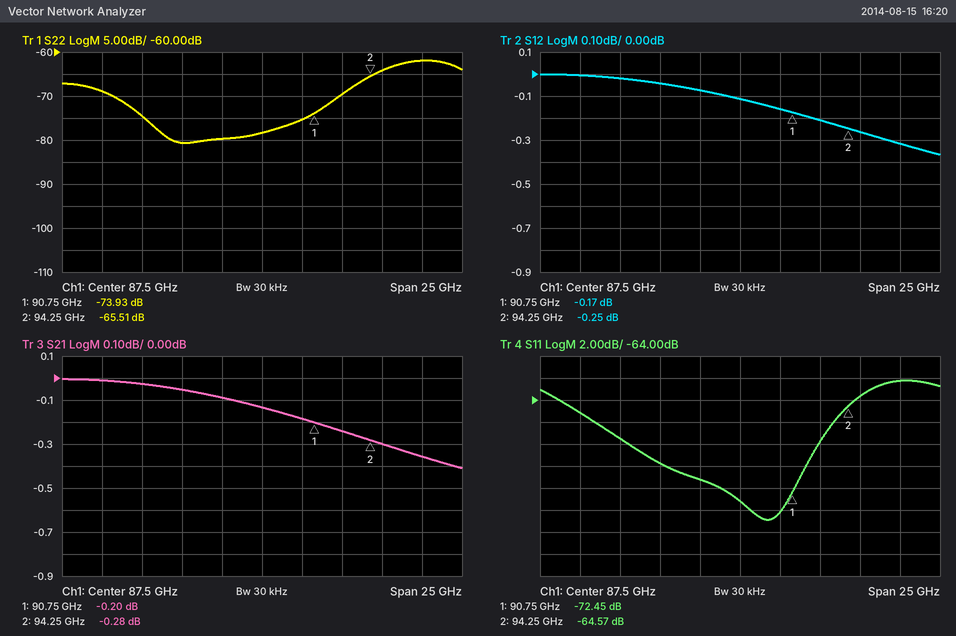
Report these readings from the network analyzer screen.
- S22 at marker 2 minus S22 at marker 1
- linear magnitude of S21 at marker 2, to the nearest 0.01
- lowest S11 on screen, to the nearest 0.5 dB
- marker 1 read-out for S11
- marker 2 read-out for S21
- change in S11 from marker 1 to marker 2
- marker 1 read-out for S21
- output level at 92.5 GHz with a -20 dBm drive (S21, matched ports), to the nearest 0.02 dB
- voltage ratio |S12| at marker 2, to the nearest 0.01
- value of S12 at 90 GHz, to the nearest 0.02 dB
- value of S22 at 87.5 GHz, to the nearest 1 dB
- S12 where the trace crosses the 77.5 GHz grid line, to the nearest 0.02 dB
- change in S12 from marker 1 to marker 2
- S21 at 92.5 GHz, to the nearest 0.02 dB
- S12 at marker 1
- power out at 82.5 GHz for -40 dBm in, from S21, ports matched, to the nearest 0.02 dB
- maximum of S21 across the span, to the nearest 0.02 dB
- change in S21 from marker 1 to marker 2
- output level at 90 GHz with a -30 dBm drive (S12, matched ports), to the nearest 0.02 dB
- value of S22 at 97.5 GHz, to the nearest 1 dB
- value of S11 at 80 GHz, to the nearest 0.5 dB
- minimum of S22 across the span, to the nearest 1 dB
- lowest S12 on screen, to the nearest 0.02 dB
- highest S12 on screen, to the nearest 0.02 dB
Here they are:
8.42 dB
0.97
-75.0 dB
-72.45 dB
-0.28 dB
7.88 dB
-0.20 dB
-20.24 dBm
0.97
-0.16 dB
-78 dB
0.00 dB
-0.08 dB
-0.24 dB
-0.17 dB
-40.06 dBm
0.00 dB
-0.08 dB
-30.16 dBm
-62 dB
-67.5 dB
-81 dB
-0.36 dB
0.00 dB
